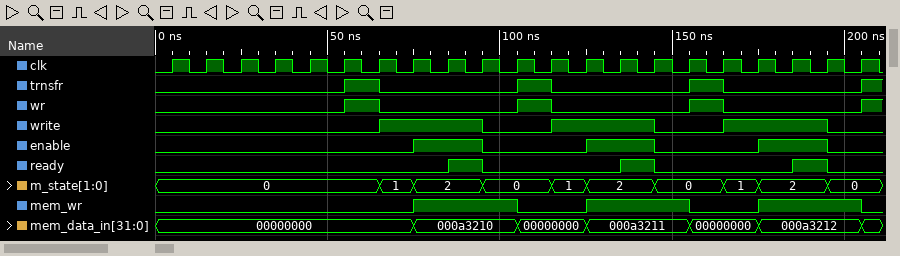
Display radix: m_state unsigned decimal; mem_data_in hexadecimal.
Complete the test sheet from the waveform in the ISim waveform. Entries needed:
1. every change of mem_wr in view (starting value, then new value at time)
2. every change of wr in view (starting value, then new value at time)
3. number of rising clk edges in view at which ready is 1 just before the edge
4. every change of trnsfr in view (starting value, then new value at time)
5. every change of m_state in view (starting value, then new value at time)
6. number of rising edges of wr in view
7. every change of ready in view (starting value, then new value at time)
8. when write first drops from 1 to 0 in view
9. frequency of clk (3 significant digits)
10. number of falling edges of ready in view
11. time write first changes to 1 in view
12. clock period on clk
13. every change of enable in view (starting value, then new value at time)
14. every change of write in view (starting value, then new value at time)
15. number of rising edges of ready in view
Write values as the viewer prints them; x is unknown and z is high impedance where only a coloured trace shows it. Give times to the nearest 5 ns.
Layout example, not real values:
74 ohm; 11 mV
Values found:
0, 1 at 75 ns, 0 at 105 ns, 1 at 125 ns, 0 at 155 ns, 1 at 175 ns, 0 at 205 ns; 0, 1 at 55 ns, 0 at 65 ns, 1 at 105 ns, 0 at 115 ns, 1 at 155 ns, 0 at 165 ns, 1 at 205 ns; 3; 0, 1 at 55 ns, 0 at 65 ns, 1 at 105 ns, 0 at 115 ns, 1 at 155 ns, 0 at 165 ns, 1 at 205 ns; 0, 1 at 65 ns, 2 at 75 ns, 0 at 95 ns, 1 at 115 ns, 2 at 125 ns, 0 at 145 ns, 1 at 165 ns, 2 at 175 ns, 0 at 195 ns; 4; 0, 1 at 85 ns, 0 at 95 ns, 1 at 135 ns, 0 at 145 ns, 1 at 185 ns, 0 at 195 ns; 95 ns; 100 MHz; 3; 65 ns; 10 ns; 0, 1 at 75 ns, 0 at 95 ns, 1 at 125 ns, 0 at 145 ns, 1 at 175 ns, 0 at 195 ns; 0, 1 at 65 ns, 0 at 95 ns, 1 at 115 ns, 0 at 145 ns, 1 at 165 ns, 0 at 195 ns; 3
